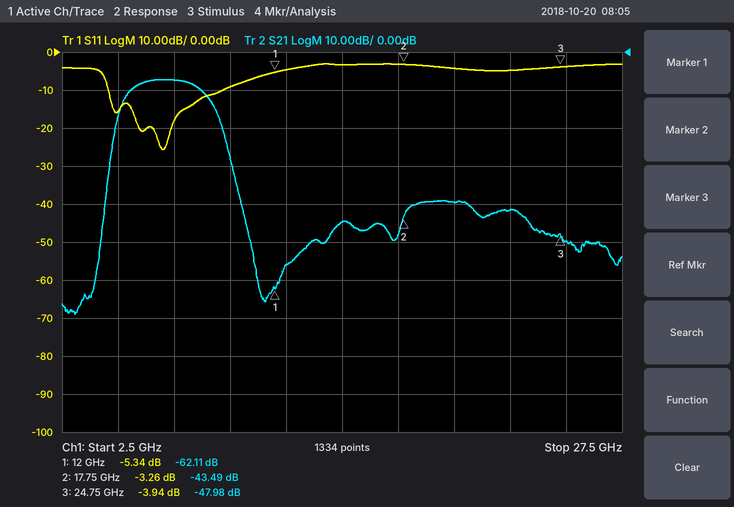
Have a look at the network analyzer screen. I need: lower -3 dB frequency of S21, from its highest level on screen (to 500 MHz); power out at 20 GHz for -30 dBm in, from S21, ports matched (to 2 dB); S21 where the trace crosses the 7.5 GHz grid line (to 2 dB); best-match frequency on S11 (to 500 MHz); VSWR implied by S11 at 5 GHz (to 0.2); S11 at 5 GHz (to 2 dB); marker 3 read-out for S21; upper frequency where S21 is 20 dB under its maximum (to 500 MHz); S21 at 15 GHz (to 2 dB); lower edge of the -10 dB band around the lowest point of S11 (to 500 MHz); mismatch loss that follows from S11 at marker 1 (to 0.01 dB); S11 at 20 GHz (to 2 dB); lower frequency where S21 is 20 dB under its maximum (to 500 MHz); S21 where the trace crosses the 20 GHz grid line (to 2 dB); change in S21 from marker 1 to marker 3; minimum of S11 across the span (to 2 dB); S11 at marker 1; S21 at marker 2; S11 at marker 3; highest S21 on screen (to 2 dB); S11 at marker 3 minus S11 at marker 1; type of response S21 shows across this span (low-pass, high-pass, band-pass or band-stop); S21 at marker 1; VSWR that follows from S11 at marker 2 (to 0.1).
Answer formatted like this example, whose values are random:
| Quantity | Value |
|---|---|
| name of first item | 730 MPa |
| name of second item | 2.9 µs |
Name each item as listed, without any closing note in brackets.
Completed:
| Quantity | Value |
|---|---|
| lower -3 dB frequency of S21, from its highest level on screen | 5.5 GHz |
| power out at 20 GHz for -30 dBm in, from S21, ports matched | -70 dBm |
| S21 where the trace crosses the 7.5 GHz grid line | -8 dB |
| best-match frequency on S11 | 7.0 GHz |
| VSWR implied by S11 at 5 GHz | 1.4 |
| S11 at 5 GHz | -16 dB |
| marker 3 read-out for S21 | -47.98 dB |
| upper frequency where S21 is 20 dB under its maximum | 10.0 GHz |
| S21 at 15 GHz | -44 dB |
| lower edge of the -10 dB band around the lowest point of S11 | 4.5 GHz |
| mismatch loss that follows from S11 at marker 1 | 1.50 dB |
| S11 at 20 GHz | -4 dB |
| lower frequency where S21 is 20 dB under its maximum | 4.5 GHz |
| S21 where the trace crosses the 20 GHz grid line | -40 dB |
| change in S21 from marker 1 to marker 3 | 14.13 dB |
| minimum of S11 across the span | -26 dB |
| S11 at marker 1 | -5.34 dB |
| S21 at marker 2 | -43.49 dB |
| S11 at marker 3 | -3.94 dB |
| highest S21 on screen | -8 dB |
| S11 at marker 3 minus S11 at marker 1 | 1.40 dB |
| type of response S21 shows across this span | band-pass |
| S21 at marker 1 | -62.11 dB |
| VSWR that follows from S11 at marker 2 | 5.4 |
